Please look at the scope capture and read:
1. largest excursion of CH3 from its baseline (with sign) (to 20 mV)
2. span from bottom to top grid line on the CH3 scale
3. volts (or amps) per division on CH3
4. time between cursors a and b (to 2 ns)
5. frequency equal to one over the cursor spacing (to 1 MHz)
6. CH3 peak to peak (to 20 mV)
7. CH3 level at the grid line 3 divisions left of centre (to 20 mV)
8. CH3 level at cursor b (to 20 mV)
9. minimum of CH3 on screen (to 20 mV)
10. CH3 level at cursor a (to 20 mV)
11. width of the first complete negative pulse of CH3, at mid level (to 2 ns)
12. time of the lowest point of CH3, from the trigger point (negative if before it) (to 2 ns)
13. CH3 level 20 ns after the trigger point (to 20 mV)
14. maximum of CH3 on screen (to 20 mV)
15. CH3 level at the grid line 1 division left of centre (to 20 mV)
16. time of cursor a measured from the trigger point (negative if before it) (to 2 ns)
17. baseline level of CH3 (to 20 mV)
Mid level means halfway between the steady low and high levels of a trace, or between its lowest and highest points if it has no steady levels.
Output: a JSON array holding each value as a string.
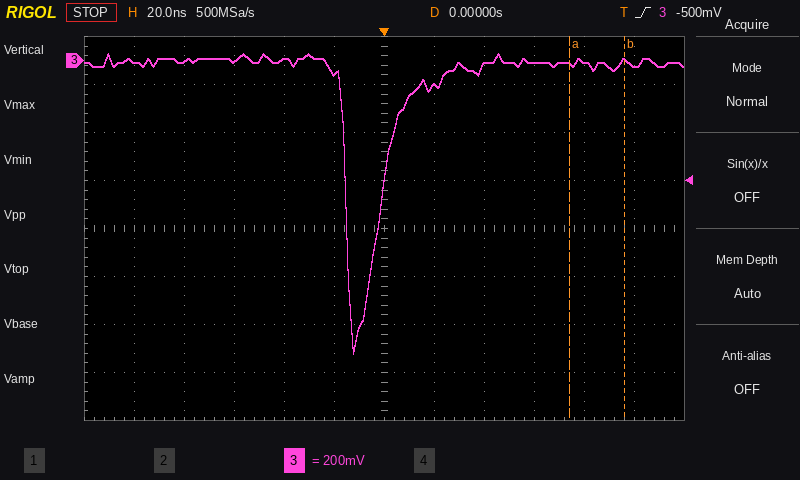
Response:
["-1.22 V", "1.6 V", "200 mV", "22 ns", "45 MHz", "1.24 V", "0 mV", "0 mV", "-1.22 V", "-20 mV", "14 ns", "-12 ns", "-100 mV", "20 mV", "-60 mV", "+74 ns", "0 mV"]
